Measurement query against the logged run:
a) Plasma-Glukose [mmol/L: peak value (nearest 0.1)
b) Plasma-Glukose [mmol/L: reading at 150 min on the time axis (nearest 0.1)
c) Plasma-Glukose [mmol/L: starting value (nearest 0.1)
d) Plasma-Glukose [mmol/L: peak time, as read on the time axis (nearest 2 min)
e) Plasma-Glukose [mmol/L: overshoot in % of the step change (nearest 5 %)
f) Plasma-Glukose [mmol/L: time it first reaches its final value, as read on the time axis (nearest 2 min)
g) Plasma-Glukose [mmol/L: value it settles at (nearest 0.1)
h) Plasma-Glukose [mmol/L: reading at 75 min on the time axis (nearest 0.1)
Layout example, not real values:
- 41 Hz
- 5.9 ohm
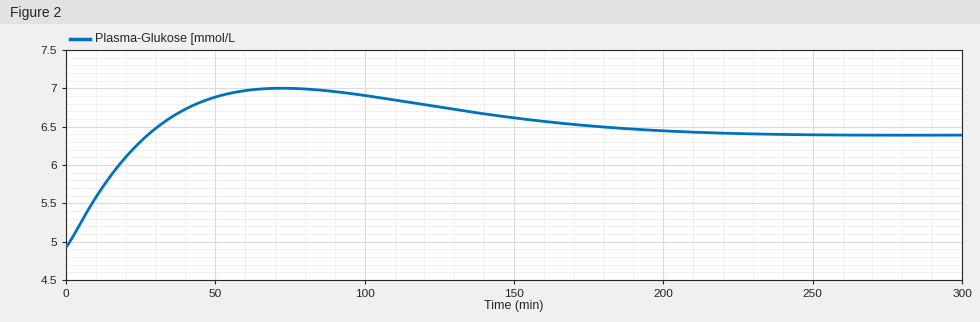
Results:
- 7.0
- 6.6
- 4.9
- 72 min
- 40 %
- 28 min
- 6.4
- 7.0
